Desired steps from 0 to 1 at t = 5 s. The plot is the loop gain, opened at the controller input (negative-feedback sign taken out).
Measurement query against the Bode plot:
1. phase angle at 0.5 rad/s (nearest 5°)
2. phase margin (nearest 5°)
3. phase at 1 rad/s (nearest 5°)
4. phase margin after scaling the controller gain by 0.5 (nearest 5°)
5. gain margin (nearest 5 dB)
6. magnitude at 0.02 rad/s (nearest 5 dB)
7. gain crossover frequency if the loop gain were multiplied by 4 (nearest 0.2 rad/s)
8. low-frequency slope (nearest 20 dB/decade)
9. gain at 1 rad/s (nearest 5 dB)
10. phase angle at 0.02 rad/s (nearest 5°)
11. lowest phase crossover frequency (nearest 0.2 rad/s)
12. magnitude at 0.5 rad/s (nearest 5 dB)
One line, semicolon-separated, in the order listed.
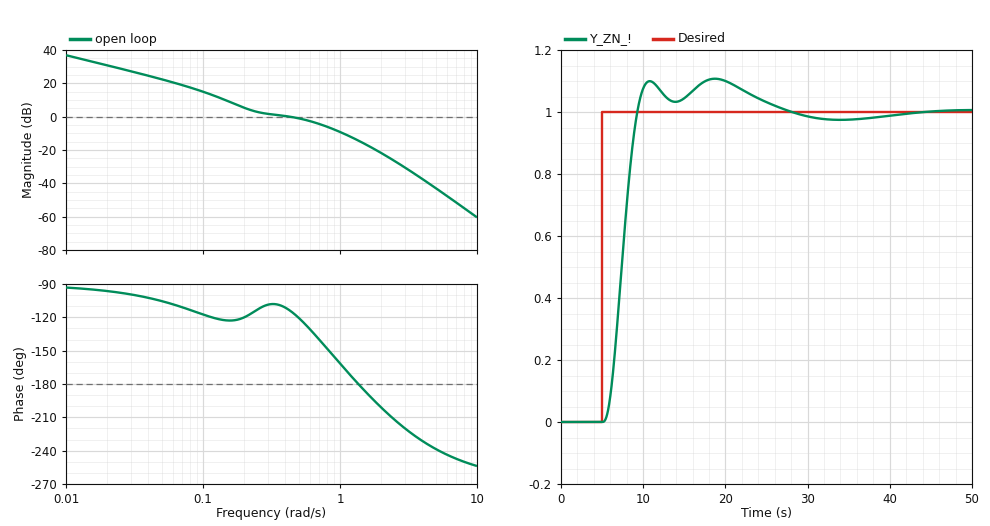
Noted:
-120°; 65°; -160°; 60°; 15 dB; 30 dB; 1.2 rad/s; -20 dB/decade; -10 dB; -95°; 1.4 rad/s; 0 dB
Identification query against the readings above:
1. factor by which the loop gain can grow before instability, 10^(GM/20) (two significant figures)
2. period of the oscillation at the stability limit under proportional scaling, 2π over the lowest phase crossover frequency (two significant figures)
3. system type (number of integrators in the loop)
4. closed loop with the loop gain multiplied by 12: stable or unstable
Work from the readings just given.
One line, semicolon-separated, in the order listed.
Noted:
5.6; 4.5 s; 1; unstable
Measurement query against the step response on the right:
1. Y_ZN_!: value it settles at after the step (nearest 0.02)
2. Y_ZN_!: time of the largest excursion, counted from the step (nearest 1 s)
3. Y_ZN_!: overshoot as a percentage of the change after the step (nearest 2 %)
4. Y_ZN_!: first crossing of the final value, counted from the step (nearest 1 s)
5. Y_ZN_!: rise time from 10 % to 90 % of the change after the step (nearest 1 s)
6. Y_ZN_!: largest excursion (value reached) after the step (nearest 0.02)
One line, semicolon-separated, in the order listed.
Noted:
1.00; 14 s; 10 %; 4 s; 3 s; 1.10
